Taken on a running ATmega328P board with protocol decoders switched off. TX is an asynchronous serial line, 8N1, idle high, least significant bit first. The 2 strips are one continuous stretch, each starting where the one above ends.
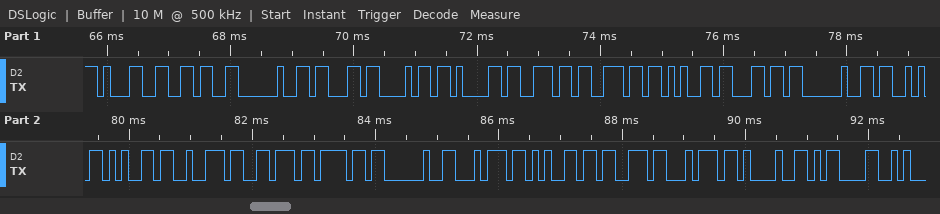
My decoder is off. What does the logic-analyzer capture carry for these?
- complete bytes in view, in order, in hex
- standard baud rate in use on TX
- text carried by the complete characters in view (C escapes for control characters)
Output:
31 36 20 63 68 61 6E 6E 65 6C 20 53 65 72 76 6F 20 74 65 73 74 21 0D
9600 baud
"16 channel Servo test!\r"
